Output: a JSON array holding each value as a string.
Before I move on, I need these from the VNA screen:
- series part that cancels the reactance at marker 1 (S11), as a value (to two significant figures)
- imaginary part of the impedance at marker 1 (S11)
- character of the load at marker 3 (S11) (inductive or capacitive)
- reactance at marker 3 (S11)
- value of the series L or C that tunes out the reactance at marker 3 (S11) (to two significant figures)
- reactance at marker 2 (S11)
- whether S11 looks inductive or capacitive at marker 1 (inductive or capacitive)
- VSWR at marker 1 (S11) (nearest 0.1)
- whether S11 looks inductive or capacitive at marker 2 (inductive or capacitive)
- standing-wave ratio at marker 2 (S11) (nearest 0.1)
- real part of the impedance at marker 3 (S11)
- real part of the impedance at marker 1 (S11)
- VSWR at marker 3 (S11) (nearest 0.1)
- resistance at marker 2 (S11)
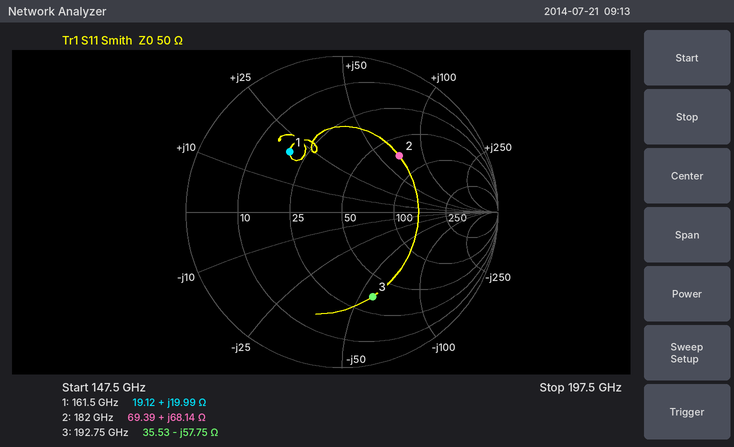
["49 fF", "+19.99 Ω", "capacitive", "-57.75 Ω", "48 pH", "+68.14 Ω", "inductive", "3.1", "inductive", "3.1", "35.53 Ω", "19.12 Ω", "3.7", "69.39 Ω"]
